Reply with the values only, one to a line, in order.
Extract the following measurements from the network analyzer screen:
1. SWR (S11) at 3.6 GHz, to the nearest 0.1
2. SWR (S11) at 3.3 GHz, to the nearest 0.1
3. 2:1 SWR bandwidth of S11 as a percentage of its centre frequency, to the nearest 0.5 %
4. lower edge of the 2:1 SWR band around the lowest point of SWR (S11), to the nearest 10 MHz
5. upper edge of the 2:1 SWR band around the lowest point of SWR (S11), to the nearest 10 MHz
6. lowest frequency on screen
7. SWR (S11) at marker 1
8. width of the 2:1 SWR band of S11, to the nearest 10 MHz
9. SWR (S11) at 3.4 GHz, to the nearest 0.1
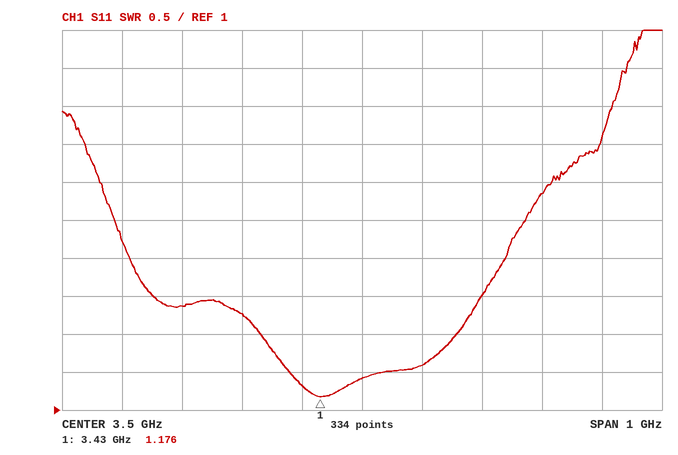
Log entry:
1.6
2.3
9.5 %
3.33 GHz
3.66 GHz
3 GHz
1.176
330 MHz
1.3
